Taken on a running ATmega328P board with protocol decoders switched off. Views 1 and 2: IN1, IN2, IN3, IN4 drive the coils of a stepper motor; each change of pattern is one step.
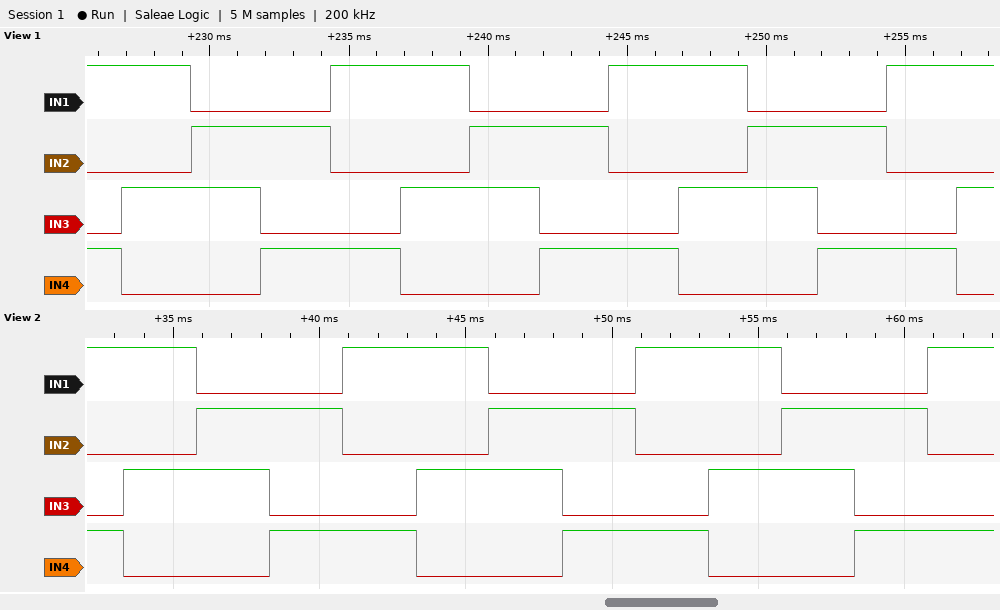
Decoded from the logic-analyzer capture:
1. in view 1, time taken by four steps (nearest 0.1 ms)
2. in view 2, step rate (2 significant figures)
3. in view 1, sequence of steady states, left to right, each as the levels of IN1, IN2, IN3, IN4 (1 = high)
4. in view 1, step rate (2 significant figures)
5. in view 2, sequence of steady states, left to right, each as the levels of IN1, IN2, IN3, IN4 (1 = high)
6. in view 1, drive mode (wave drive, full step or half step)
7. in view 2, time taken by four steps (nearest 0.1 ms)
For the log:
10.0 ms
400 steps/s
1001 1010 0110 0101 1001 1010 0110 0101 1001 1010 0110 0101 1001 1010
400 steps/s
1001 1010 0110 0101 1001 1010 0110 0101 1001 1010 0110 0101 1001
full step
10.0 ms
